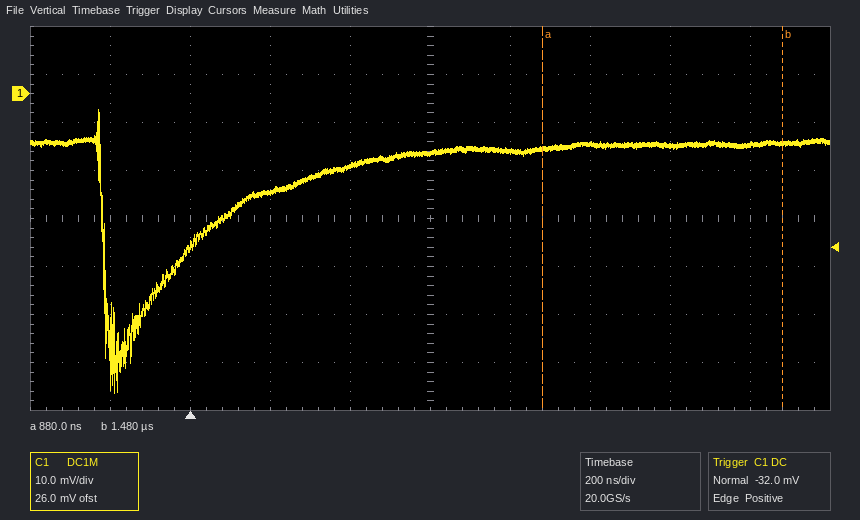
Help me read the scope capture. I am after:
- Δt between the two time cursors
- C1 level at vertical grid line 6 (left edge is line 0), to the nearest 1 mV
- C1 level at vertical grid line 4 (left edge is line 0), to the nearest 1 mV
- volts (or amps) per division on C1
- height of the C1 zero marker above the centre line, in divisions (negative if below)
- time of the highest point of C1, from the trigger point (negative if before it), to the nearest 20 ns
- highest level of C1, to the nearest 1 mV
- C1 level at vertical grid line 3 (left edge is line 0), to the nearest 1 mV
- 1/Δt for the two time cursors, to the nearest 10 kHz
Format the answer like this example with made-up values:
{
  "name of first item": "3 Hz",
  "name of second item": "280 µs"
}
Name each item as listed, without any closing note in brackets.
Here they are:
{
  "Δt between the two time cursors": "600 ns",
  "C1 level at vertical grid line 6 (left edge is line 0), to the nearest 1 mV": "-12 mV",
  "C1 level at vertical grid line 4 (left edge is line 0), to the nearest 1 mV": "-15 mV",
  "volts (or amps) per division on C1": "10 mV",
  "height of the C1 zero marker above the centre line, in divisions": "+2.6 div",
  "time of the highest point of C1, from the trigger point (negative if before it), to the nearest 20 ns": "-220 ns",
  "highest level of C1, to the nearest 1 mV": "-3 mV",
  "C1 level at vertical grid line 3 (left edge is line 0), to the nearest 1 mV": "-21 mV",
  "1/Δt for the two time cursors, to the nearest 10 kHz": "1.67 MHz"
}
